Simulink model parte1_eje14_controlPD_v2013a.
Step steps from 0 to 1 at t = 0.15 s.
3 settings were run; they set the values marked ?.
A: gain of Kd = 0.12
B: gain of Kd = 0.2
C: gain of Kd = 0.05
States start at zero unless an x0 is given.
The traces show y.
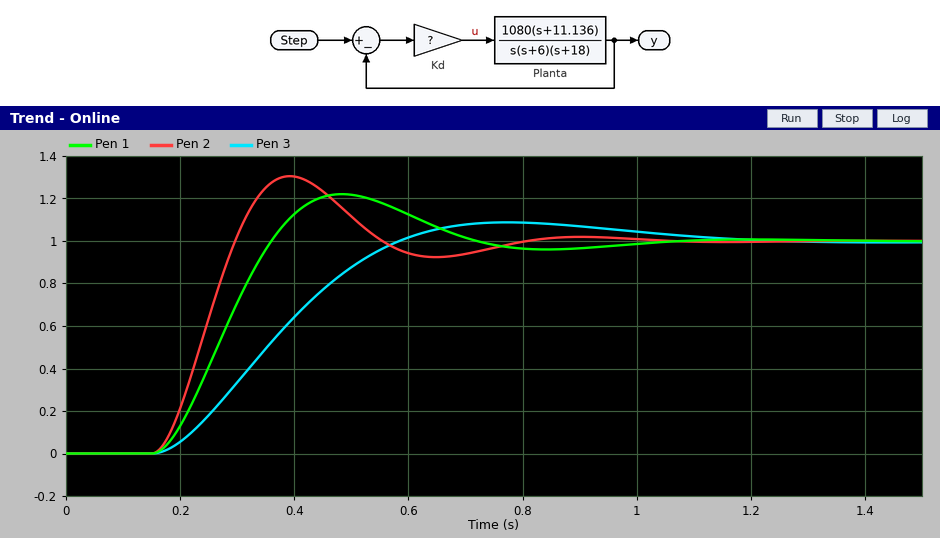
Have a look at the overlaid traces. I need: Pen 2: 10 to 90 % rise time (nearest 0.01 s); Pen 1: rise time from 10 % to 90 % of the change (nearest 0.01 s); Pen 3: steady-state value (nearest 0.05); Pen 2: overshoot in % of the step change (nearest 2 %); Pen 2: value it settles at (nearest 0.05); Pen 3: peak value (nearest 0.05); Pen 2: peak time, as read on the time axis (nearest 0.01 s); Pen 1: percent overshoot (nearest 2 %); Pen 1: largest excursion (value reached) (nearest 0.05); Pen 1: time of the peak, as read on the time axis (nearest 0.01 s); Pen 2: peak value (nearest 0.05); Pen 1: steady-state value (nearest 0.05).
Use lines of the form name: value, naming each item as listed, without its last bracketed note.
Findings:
Pen 2: 10 to 90 % rise time: 0.10 s
Pen 1: rise time from 10 % to 90 % of the change: 0.14 s
Pen 3: steady-state value: 1.00
Pen 2: overshoot in % of the step change: 30 %
Pen 2: value it settles at: 1.00
Pen 3: peak value: 1.10
Pen 2: peak time, as read on the time axis: 0.39 s
Pen 1: percent overshoot: 22 %
Pen 1: largest excursion (value reached): 1.20
Pen 1: time of the peak, as read on the time axis: 0.48 s
Pen 2: peak value: 1.30
Pen 1: steady-state value: 1.00
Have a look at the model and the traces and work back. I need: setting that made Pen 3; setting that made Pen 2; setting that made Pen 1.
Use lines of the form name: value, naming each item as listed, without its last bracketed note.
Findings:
setting that made Pen 3: C
setting that made Pen 2: B
setting that made Pen 1: A
